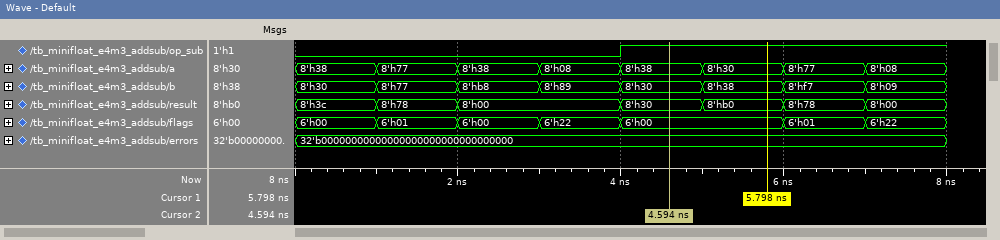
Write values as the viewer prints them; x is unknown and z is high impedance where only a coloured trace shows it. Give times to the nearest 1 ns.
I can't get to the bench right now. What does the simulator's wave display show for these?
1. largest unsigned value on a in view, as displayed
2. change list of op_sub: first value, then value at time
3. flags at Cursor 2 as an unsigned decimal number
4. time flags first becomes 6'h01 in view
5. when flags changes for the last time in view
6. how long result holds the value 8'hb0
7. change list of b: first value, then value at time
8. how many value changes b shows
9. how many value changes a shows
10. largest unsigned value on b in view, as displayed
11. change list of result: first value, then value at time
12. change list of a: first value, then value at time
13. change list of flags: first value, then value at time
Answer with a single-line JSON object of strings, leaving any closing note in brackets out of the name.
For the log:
{"largest unsigned value on a in view, as displayed": "8'h77", "change list of op_sub: first value, then value at time": "0, 1 at 4 ns", "flags at Cursor 2 as an unsigned decimal number": "0", "time flags first becomes 6'h01 in view": "1 ns", "when flags changes for the last time in view": "7 ns", "how long result holds the value 8'hb0": "1 ns", "change list of b: first value, then value at time": "8'h30, 8'h77 at 1 ns, 8'hb8 at 2 ns, 8'h89 at 3 ns, 8'h30 at 4 ns, 8'h38 at 5 ns, 8'hf7 at 6 ns, 8'h09 at 7 ns", "how many value changes b shows": "7", "how many value changes a shows": "7", "largest unsigned value on b in view, as displayed": "8'hf7", "change list of result: first value, then value at time": "8'h3c, 8'h78 at 1 ns, 8'h00 at 2 ns, 8'h30 at 4 ns, 8'hb0 at 5 ns, 8'h78 at 6 ns, 8'h00 at 7 ns", "change list of a: first value, then value at time": "8'h38, 8'h77 at 1 ns, 8'h38 at 2 ns, 8'h08 at 3 ns, 8'h38 at 4 ns, 8'h30 at 5 ns, 8'h77 at 6 ns, 8'h08 at 7 ns", "change list of flags: first value, then value at time": "6'h00, 6'h01 at 1 ns, 6'h00 at 2 ns, 6'h22 at 3 ns, 6'h00 at 4 ns, 6'h01 at 6 ns, 6'h22 at 7 ns"}
